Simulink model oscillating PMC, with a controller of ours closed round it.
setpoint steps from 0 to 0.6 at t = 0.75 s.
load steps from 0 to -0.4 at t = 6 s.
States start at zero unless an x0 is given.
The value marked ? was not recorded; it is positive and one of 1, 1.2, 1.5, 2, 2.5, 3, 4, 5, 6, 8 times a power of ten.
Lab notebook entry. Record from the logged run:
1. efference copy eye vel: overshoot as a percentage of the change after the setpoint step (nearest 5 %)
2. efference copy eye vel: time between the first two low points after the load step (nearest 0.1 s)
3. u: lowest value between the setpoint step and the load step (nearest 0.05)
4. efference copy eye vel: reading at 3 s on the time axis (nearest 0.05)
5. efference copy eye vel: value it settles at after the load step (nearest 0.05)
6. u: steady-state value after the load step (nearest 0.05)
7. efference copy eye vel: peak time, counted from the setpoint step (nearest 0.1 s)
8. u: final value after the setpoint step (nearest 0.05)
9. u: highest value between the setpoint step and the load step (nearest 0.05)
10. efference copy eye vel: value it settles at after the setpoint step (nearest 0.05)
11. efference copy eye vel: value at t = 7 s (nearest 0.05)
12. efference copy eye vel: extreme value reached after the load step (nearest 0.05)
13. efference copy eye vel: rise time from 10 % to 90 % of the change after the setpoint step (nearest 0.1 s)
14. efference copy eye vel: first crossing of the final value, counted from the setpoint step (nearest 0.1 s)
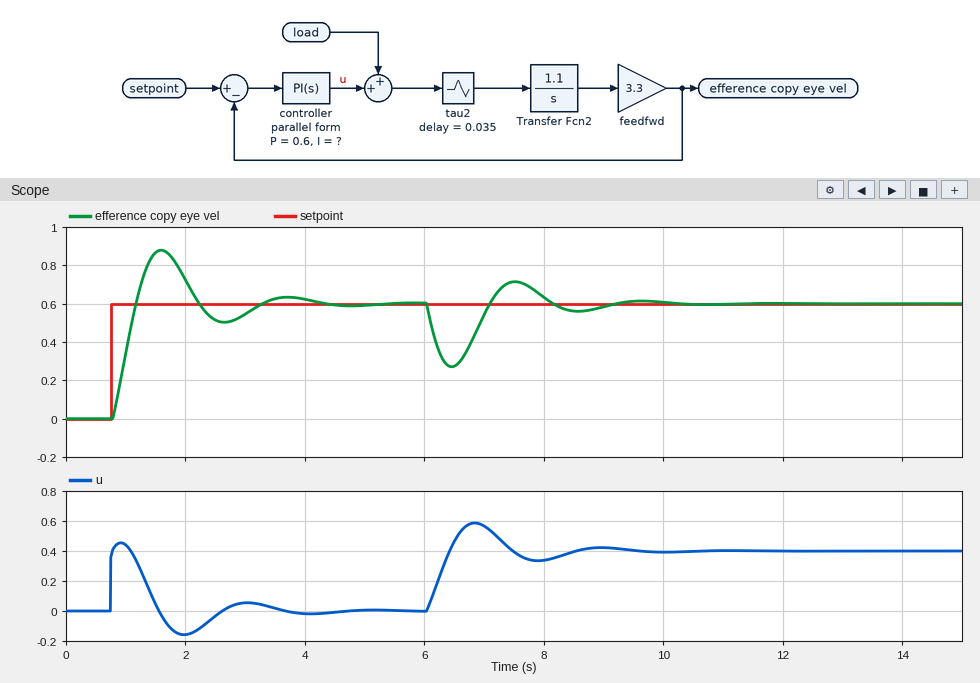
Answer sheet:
45 %
2.1 s
-0.15
0.55
0.60
0.40
0.8 s
0.00
0.45
0.60
0.55
0.25
0.3 s
0.4 s
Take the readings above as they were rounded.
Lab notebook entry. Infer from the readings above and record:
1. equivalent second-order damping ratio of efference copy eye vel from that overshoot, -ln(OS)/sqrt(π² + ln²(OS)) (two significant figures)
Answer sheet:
0.25
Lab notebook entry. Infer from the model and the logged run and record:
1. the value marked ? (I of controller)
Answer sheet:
2.5
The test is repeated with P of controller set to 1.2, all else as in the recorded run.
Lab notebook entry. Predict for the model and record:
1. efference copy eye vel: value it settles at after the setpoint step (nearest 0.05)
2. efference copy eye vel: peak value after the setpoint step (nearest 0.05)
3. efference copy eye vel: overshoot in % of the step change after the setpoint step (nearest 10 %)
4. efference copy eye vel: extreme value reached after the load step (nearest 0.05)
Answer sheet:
0.60
0.75
20 %
0.35
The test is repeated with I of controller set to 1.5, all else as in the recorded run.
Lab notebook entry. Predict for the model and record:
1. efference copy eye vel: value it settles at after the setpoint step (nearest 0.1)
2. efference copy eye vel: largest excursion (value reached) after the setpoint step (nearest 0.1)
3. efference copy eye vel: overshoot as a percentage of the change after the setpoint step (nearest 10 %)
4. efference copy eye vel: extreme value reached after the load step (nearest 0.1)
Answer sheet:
0.6
0.8
40 %
0.2
